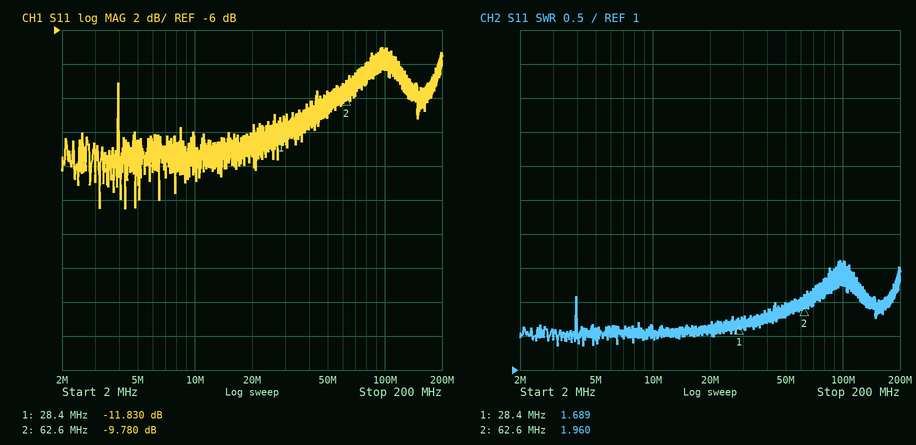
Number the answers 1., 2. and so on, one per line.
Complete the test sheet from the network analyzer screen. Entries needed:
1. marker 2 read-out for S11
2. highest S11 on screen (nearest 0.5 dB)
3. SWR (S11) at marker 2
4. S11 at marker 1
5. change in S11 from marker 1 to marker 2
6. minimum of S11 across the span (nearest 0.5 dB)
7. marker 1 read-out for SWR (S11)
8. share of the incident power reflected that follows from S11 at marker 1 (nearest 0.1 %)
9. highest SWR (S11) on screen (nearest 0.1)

1. -9.780 dB
2. -7.0 dB
3. 1.960
4. -11.830 dB
5. 2.050 dB
6. -16.5 dB
7. 1.689
8. 6.6 %
9. 2.6
